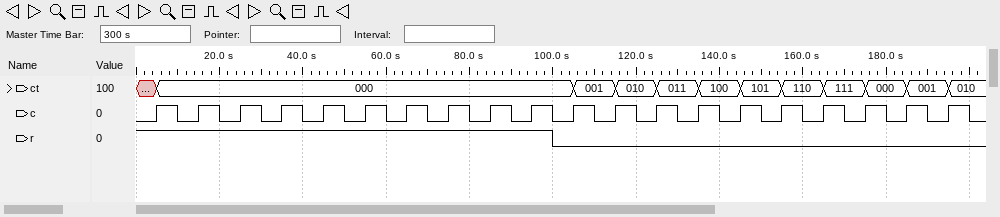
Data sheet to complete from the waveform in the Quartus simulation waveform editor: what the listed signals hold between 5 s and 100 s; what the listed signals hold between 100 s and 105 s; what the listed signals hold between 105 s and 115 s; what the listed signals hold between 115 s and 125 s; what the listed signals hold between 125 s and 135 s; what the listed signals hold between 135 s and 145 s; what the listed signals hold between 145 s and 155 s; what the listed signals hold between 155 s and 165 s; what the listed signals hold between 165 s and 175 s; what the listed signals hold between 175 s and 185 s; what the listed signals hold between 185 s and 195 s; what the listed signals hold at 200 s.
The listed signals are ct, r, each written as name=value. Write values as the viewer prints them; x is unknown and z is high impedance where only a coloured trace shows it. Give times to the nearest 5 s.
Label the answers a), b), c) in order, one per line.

a) ct=000, r=1
b) ct=000, r=0
c) ct=001, r=0
d) ct=010, r=0
e) ct=011, r=0
f) ct=100, r=0
g) ct=101, r=0
h) ct=110, r=0
i) ct=111, r=0
j) ct=000, r=0
k) ct=001, r=0
l) ct=010, r=0
